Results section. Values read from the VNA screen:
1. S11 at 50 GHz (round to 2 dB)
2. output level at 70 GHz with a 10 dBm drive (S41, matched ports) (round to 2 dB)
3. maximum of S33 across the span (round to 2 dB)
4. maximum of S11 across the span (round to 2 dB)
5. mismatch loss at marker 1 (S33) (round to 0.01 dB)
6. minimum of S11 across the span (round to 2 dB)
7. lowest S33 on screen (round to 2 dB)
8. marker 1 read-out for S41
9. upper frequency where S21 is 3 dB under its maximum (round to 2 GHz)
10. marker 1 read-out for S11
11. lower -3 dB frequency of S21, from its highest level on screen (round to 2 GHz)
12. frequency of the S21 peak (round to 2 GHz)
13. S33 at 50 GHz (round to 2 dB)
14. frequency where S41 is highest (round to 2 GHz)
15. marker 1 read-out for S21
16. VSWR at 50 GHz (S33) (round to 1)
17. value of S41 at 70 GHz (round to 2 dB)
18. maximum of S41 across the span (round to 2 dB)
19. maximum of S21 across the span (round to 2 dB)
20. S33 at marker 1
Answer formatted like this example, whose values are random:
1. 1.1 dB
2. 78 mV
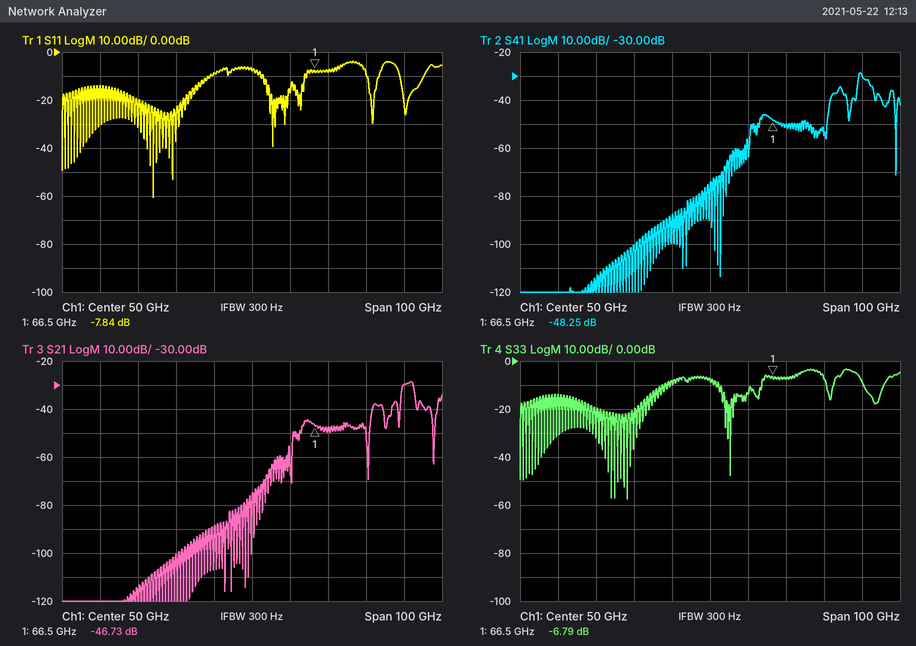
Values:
1. -8 dB
2. -40 dBm
3. -4 dB
4. -4 dB
5. 1.02 dB
6. -60 dB
7. -58 dB
8. -48.25 dB
9. 92 GHz
10. -7.84 dB
11. 90 GHz
12. 92 GHz
13. -8 dB
14. 90 GHz
15. -46.73 dB
16. 2
17. -50 dB
18. -28 dB
19. -28 dB
20. -6.79 dB
